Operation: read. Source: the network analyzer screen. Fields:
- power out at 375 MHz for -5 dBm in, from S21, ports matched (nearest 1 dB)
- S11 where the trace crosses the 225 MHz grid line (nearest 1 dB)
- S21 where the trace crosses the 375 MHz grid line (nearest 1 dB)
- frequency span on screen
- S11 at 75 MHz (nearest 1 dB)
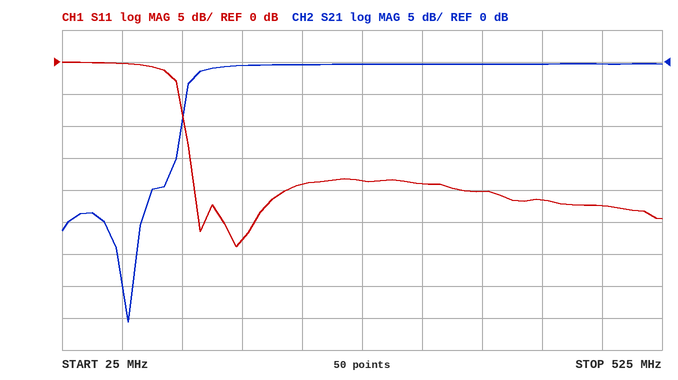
-5 dBm
-19 dB
0 dB
500 MHz
0 dB
